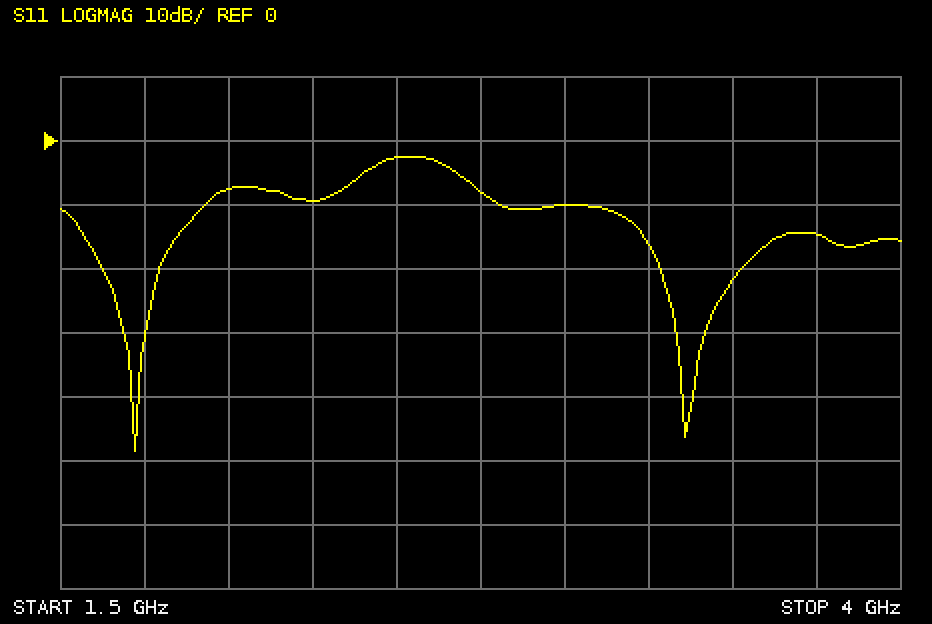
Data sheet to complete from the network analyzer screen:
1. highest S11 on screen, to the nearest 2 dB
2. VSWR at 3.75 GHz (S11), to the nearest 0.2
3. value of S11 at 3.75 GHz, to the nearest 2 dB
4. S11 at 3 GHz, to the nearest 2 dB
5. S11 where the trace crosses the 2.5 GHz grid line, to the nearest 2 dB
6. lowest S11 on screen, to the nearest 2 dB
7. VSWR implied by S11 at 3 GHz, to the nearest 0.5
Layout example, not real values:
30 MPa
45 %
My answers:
-2 dB
1.4
-14 dB
-10 dB
-2 dB
-48 dB
2.0
